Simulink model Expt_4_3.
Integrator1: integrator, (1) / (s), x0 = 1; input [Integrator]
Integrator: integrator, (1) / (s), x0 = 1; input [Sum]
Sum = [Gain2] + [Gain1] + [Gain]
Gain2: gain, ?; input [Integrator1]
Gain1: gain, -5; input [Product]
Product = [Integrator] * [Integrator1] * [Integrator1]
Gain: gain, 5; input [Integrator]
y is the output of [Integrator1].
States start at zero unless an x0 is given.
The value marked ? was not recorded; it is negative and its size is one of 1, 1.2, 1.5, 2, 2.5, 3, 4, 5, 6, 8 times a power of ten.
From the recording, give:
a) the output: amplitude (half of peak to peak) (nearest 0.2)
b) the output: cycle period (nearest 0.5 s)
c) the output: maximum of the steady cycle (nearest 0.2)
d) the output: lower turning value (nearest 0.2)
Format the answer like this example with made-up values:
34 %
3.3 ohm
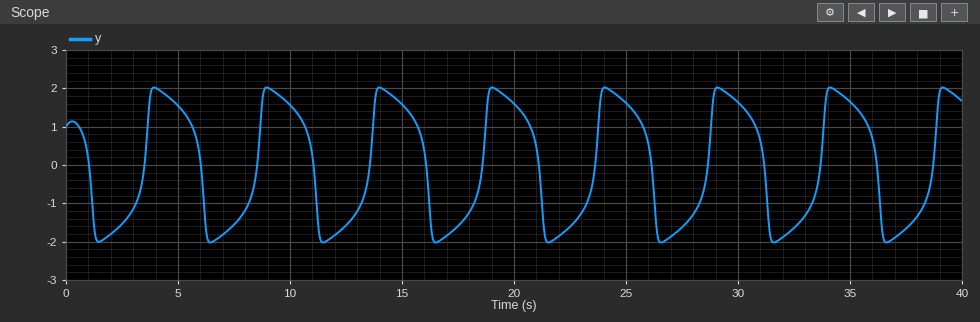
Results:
2.0
5.0 s
2.0
-2.0
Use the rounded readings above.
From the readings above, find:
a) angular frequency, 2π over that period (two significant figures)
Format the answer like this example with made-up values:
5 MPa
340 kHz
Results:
1.3 rad/s
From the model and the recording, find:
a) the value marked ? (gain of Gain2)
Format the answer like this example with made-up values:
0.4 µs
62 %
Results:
-3
